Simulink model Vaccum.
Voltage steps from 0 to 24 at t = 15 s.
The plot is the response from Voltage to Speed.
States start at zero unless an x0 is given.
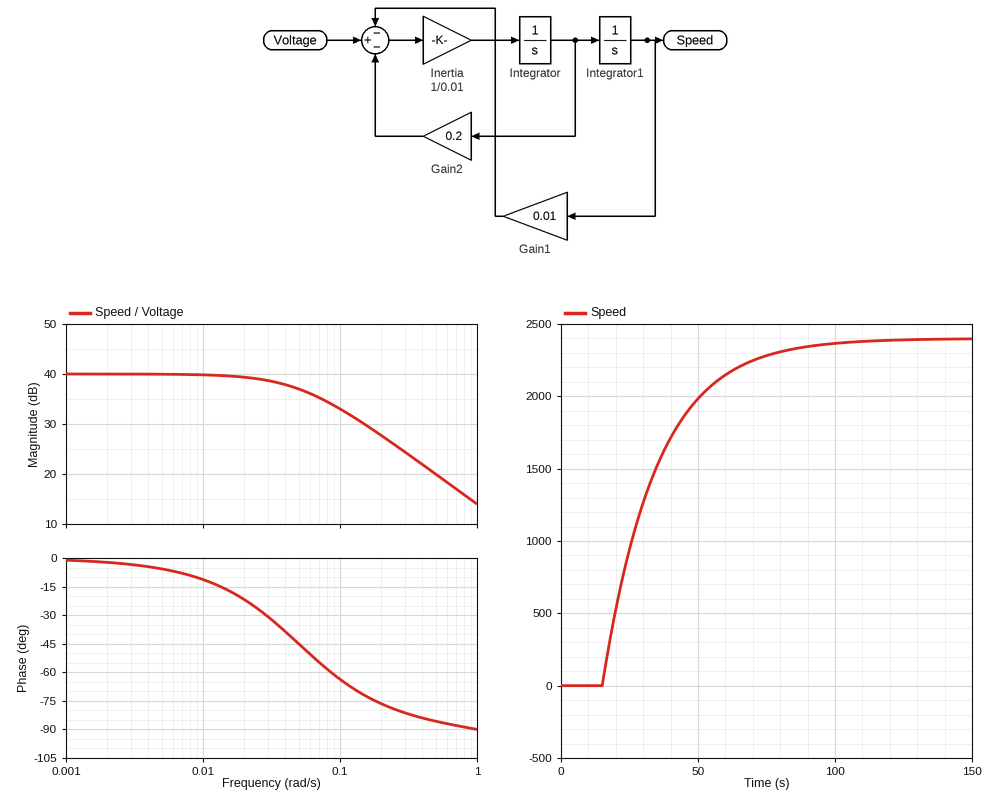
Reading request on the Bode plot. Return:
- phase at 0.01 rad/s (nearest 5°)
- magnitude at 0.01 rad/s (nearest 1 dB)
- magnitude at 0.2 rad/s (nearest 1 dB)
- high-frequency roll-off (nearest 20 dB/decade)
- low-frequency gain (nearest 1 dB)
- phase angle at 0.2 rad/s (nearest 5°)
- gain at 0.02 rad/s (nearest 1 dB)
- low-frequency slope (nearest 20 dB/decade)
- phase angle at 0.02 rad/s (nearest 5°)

-10°
40 dB
28 dB
-20 dB/decade
40 dB
-75°
39 dB
0 dB/decade
-20°
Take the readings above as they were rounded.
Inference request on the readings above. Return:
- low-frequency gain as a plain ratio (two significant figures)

100
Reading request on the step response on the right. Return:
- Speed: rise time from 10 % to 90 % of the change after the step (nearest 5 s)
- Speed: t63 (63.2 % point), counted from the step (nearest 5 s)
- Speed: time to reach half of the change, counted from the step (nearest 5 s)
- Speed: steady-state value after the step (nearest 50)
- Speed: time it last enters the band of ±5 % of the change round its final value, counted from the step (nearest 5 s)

45 s
20 s
15 s
2400
60 s
